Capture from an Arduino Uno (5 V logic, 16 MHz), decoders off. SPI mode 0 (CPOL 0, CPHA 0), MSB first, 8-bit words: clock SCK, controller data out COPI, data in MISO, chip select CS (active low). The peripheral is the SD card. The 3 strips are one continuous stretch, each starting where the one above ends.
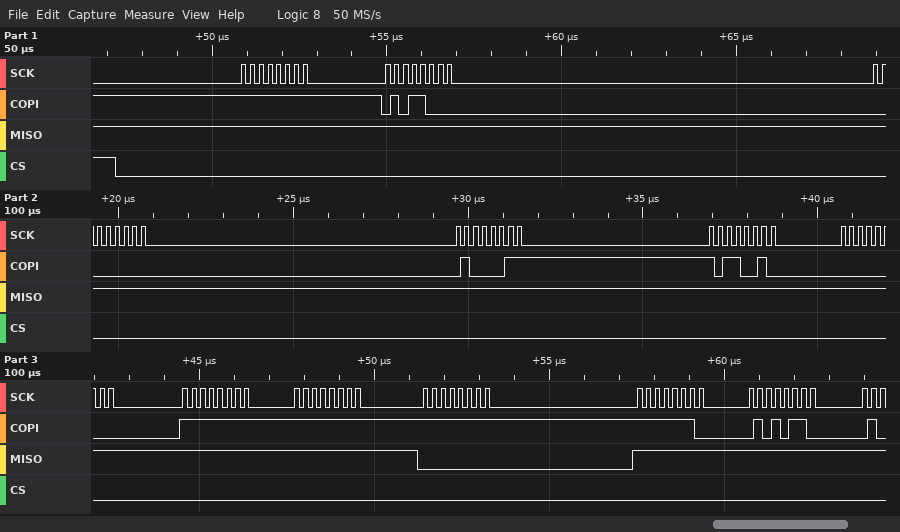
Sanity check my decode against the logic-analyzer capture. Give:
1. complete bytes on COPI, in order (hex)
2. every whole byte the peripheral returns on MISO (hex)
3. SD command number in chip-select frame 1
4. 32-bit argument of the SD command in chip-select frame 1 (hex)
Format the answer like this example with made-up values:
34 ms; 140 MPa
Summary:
0xFF 0x58 0x00 0x43 0xB2 0x00 0xFF 0xFF 0xFF 0xFE 0x56; 0xFF 0xFF 0xFF 0xFF 0xFF 0xFF 0xFF 0xFF 0x00 0xFF 0xFF; CMD24; 0x0043B200
